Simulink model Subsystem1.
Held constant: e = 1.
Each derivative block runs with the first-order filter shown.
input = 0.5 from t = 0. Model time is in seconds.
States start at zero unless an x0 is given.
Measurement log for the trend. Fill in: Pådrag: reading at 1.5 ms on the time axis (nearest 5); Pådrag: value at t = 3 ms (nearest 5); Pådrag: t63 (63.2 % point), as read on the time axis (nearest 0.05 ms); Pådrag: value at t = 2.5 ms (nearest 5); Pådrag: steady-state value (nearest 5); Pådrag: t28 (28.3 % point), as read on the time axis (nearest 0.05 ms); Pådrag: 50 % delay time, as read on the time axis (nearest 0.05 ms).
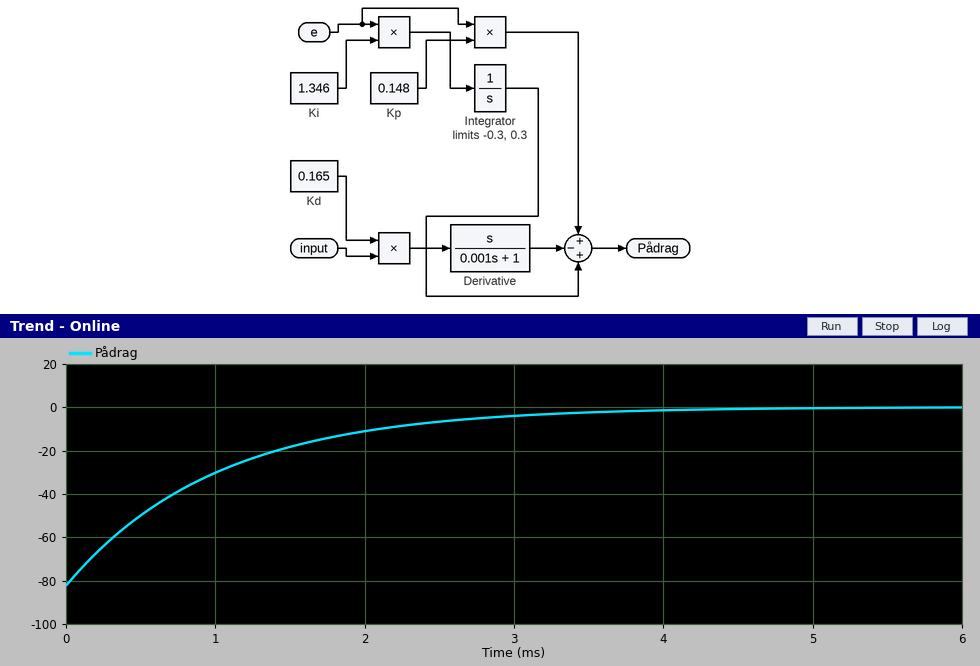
-20
-5
1.00 ms
-5
0
0.35 ms
0.70 ms
